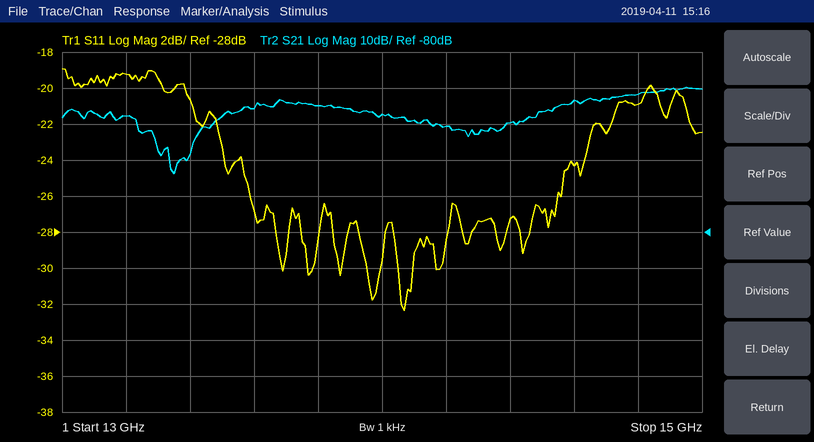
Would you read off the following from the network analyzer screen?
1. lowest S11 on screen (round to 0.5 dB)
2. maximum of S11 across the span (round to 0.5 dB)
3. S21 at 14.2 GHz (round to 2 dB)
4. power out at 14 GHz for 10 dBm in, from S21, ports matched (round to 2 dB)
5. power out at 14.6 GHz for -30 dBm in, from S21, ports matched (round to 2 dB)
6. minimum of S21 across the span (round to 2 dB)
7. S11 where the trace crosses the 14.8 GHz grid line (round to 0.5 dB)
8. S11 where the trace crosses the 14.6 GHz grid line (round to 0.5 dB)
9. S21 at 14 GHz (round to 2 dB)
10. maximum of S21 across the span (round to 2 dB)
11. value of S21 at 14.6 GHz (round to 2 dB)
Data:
-32.5 dB
-19.0 dB
-50 dB
-38 dBm
-74 dBm
-64 dB
-21.0 dB
-24.5 dB
-48 dB
-40 dB
-44 dB
